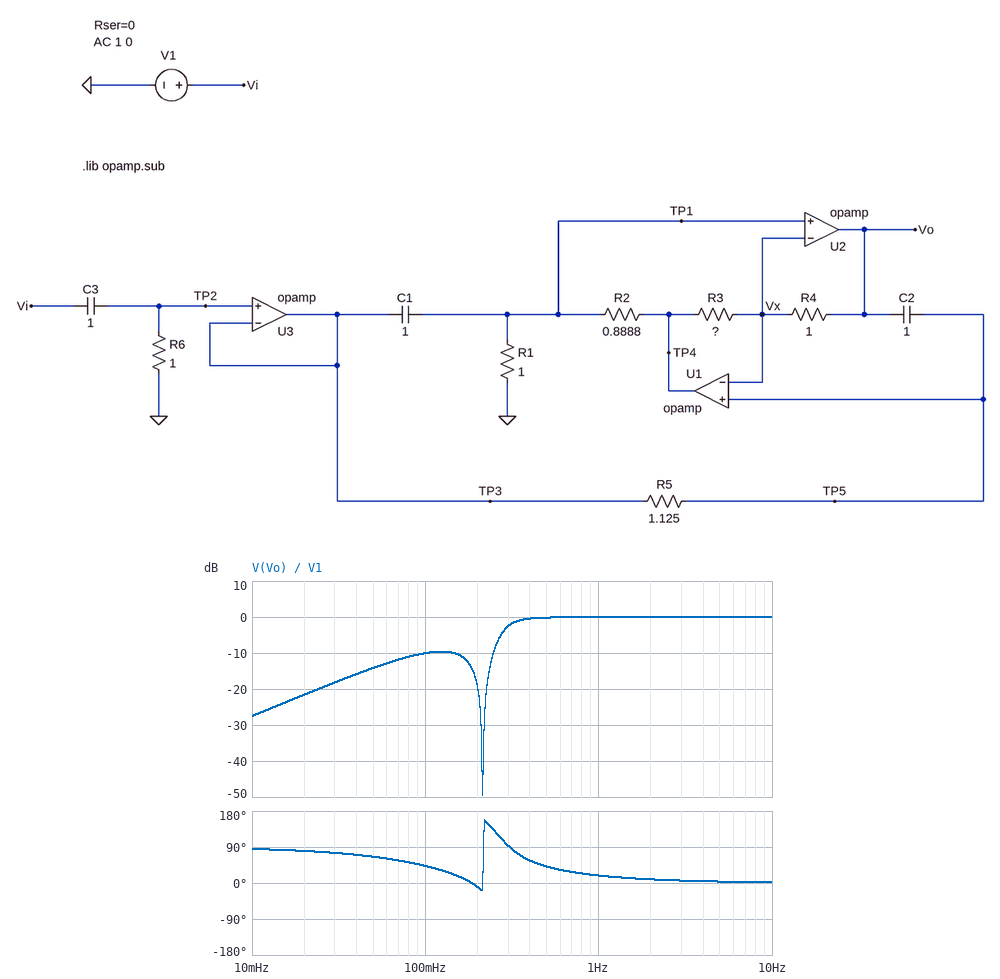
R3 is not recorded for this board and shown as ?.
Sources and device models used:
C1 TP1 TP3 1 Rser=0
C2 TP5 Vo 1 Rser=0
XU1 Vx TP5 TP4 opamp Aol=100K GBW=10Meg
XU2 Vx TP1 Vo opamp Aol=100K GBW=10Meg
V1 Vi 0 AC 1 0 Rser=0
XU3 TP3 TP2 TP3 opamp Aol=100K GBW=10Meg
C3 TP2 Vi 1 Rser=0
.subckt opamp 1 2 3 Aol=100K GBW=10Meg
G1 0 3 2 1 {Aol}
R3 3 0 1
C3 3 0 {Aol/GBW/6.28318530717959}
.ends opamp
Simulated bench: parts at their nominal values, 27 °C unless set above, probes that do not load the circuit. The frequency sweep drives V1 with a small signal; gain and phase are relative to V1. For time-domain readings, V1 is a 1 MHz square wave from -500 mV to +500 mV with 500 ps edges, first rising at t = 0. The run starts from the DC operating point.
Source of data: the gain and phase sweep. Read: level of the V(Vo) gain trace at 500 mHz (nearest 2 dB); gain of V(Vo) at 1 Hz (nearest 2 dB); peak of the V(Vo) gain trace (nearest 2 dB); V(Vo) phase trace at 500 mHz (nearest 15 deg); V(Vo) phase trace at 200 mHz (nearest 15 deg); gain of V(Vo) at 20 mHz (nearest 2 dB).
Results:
0 dB
0 dB
0 dB
45 deg
-15 deg
-22 dB
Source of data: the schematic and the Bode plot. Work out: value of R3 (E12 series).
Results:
2.7 Ω
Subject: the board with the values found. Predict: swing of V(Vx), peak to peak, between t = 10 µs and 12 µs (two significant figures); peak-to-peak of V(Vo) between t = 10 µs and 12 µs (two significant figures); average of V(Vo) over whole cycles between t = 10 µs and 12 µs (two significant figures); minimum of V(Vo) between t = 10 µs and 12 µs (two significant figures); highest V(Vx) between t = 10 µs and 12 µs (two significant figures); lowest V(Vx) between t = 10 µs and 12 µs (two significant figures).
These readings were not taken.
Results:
1.0 V
1.2 V
500 mV
-110 mV
1.0 V
-21 mV
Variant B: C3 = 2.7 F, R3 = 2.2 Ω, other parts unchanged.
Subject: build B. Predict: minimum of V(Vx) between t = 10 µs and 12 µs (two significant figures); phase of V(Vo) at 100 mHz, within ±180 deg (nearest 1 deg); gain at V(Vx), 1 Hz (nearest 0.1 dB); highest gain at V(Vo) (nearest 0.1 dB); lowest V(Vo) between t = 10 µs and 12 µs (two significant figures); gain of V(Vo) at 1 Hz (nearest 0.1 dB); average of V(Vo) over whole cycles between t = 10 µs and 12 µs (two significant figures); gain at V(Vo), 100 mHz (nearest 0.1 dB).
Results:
-25 mV
11 deg
-0.1 dB
0.2 dB
-120 mV
0.1 dB
500 mV
-7.7 dB
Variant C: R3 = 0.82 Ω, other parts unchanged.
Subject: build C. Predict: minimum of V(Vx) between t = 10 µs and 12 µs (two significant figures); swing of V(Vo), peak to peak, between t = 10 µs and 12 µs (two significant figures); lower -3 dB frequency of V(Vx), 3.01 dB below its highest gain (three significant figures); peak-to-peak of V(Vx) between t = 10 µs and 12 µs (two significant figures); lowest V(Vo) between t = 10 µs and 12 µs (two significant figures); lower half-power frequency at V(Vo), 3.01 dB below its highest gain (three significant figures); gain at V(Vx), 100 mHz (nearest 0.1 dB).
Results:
-48 mV
1.3 V
289 mHz
1.1 V
-150 mV
152 mHz
-10.5 dB
